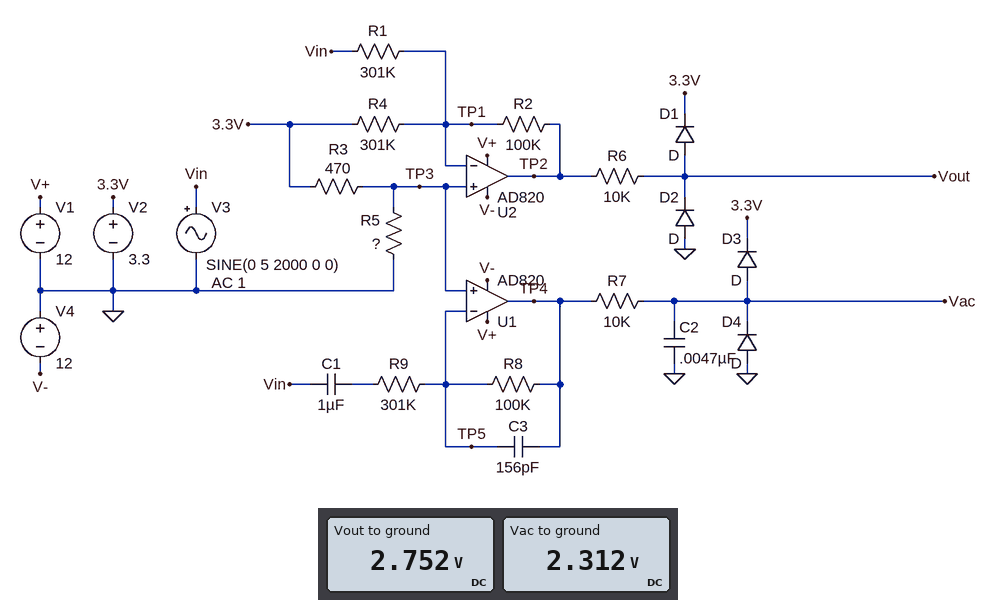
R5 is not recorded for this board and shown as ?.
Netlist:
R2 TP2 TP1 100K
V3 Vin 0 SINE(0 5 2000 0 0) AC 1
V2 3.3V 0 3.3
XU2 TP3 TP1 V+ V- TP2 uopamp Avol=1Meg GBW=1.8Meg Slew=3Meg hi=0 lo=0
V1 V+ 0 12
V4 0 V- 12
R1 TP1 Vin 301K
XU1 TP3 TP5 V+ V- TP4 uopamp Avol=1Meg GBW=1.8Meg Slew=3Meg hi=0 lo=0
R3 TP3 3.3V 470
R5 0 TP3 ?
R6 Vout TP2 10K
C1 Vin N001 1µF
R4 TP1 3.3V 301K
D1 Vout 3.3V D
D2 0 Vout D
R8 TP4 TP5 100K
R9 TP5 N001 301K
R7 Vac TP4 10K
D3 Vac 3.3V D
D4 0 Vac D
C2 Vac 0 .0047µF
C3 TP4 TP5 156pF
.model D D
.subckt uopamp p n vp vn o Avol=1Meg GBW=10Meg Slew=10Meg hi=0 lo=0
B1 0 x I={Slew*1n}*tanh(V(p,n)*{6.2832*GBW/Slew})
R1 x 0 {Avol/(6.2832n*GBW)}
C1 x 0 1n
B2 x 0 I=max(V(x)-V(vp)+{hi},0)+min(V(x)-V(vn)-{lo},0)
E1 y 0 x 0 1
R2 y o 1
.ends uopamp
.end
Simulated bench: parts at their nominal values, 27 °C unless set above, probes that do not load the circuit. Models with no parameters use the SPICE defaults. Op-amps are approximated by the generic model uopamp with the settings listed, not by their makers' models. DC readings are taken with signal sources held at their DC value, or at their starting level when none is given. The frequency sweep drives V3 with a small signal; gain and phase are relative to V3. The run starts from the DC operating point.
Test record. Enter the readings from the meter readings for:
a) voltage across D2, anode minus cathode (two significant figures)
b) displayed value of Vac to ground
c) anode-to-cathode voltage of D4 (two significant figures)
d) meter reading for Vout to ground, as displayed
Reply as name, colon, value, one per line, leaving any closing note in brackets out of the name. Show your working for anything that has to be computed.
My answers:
voltage across D2, anode minus cathode: 0 V - 2.752 V = -2.8 V
displayed value of Vac to ground: 2.312 V
anode-to-cathode voltage of D4: 0 V - 2.312 V = -2.3 V
meter reading for Vout to ground, as displayed: 2.752 V
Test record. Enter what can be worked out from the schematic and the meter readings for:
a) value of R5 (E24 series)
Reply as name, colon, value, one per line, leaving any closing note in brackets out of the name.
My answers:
value of R5: 1.1 kΩ
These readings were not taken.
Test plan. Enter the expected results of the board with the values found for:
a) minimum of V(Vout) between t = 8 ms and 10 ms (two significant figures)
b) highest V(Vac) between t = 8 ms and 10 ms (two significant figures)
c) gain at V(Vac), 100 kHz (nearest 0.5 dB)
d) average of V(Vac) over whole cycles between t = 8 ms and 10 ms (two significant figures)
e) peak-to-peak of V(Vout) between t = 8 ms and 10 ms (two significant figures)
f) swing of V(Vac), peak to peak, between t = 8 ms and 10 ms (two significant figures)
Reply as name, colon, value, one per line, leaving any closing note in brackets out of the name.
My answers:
minimum of V(Vout) between t = 8 ms and 10 ms: 1.1 V
highest V(Vac) between t = 8 ms and 10 ms: 3.7 V
gain at V(Vac), 100 kHz: -59.0 dB
average of V(Vac) over whole cycles between t = 8 ms and 10 ms: 2.3 V
peak-to-peak of V(Vout) between t = 8 ms and 10 ms: 2.8 V
swing of V(Vac), peak to peak, between t = 8 ms and 10 ms: 2.8 V
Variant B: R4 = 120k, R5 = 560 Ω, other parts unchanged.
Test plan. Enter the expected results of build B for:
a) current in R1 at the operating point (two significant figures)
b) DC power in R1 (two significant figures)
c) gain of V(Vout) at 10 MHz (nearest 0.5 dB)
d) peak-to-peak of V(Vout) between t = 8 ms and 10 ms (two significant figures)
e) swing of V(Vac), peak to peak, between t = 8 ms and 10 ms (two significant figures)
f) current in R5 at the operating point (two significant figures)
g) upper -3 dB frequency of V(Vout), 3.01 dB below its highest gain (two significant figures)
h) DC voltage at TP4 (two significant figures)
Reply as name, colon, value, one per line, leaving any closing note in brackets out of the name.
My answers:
current in R1 at the operating point: 6.0 µA
DC power in R1: 11 µW
gain of V(Vout) at 10 MHz: -31.0 dB
peak-to-peak of V(Vout) between t = 8 ms and 10 ms: 3.3 V
swing of V(Vac), peak to peak, between t = 8 ms and 10 ms: 2.8 V
current in R5 at the operating point: 3.2 mA
upper -3 dB frequency of V(Vout), 3.01 dB below its highest gain: 830 kHz
DC voltage at TP4: 1.8 V
